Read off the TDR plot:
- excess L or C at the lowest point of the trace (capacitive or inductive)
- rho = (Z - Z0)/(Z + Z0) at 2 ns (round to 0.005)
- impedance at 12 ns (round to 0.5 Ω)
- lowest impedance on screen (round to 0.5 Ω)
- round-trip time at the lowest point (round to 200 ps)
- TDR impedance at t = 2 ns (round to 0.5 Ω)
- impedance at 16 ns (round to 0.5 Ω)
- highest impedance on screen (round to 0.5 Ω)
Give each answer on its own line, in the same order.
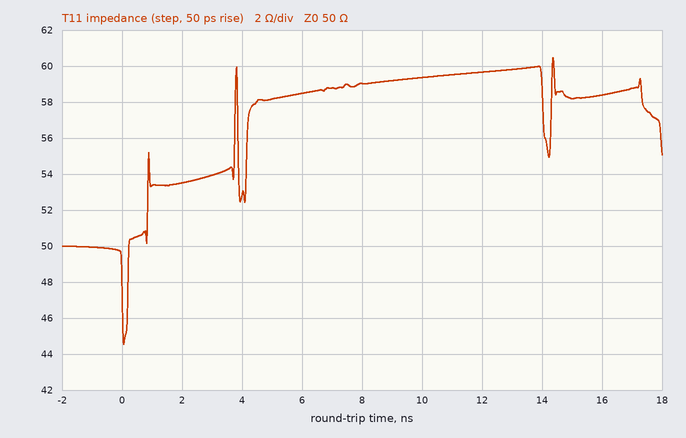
capacitive
+0.035
59.5 Ω
44.5 Ω
0.0 ns
53.5 Ω
58.5 Ω
60.5 Ω
